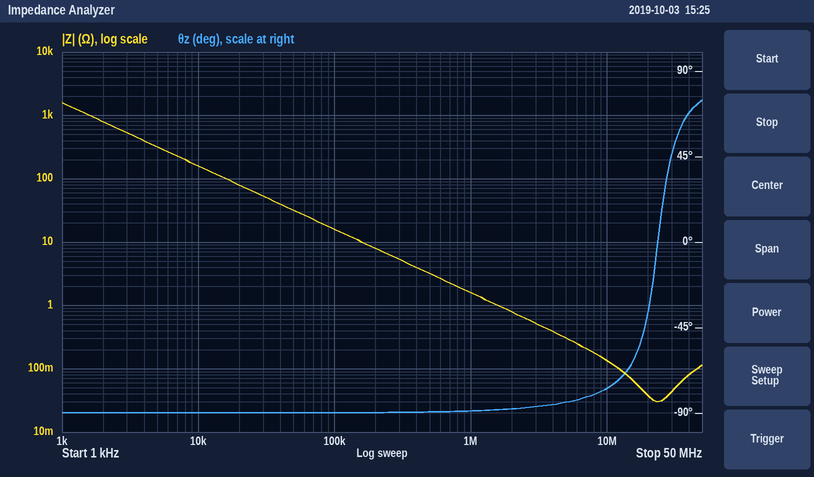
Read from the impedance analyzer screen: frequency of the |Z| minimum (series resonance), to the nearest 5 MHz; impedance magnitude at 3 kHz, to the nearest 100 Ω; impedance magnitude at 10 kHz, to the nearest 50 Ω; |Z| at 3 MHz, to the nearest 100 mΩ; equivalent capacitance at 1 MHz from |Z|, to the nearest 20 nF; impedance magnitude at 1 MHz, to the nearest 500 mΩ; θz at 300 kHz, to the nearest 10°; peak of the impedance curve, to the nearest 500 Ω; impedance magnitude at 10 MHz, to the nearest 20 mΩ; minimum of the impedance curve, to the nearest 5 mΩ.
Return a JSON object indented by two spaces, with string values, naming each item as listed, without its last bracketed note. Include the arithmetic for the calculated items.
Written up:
{
  "frequency of the |Z| minimum (series resonance), to the nearest 5 MHz": "25 MHz",
  "impedance magnitude at 3 kHz, to the nearest 100 Ω": "500 Ω",
  "impedance magnitude at 10 kHz, to the nearest 50 Ω": "150 Ω",
  "|Z| at 3 MHz, to the nearest 100 mΩ": "500 mΩ",
  "equivalent capacitance at 1 MHz from |Z|, to the nearest 20 nF": "C = 1/(2π × 1 MHz × 1.5 Ω) ≈ 106 nF, so 100 nF to the nearest 20 nF",
  "impedance magnitude at 1 MHz, to the nearest 500 mΩ": "1.5 Ω",
  "θz at 300 kHz, to the nearest 10°": "-90°",
  "peak of the impedance curve, to the nearest 500 Ω": "1.5 kΩ",
  "impedance magnitude at 10 MHz, to the nearest 20 mΩ": "140 mΩ",
  "minimum of the impedance curve, to the nearest 5 mΩ": "30 mΩ"
}
